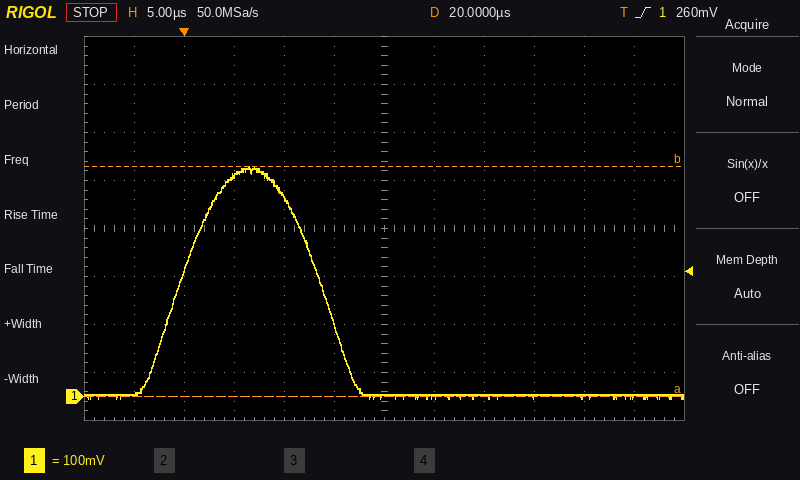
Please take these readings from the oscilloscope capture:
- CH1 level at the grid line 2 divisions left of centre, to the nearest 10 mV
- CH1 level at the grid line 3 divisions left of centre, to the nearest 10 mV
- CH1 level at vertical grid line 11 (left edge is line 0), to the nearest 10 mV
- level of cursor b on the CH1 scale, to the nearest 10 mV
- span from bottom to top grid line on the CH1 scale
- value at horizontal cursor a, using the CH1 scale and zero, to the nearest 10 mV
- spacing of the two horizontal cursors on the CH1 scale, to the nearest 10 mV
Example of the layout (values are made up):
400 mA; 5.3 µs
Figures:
410 mV; 460 mV; 0 mV; 480 mV; 800 mV; 0 mV; 480 mV
